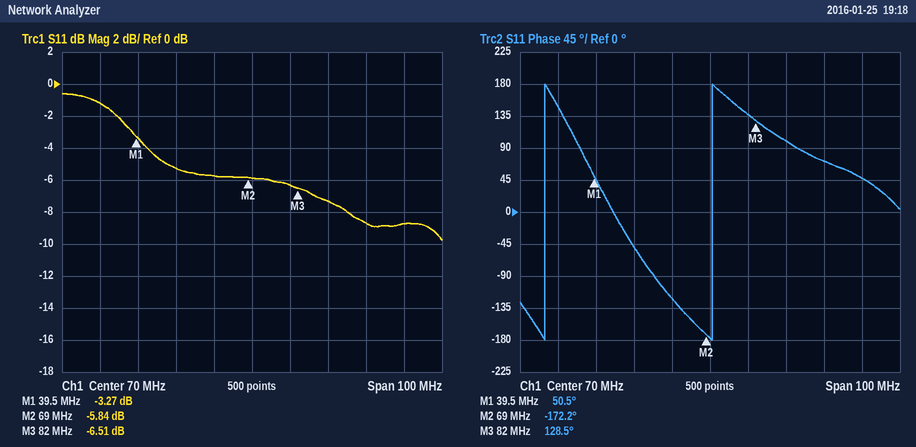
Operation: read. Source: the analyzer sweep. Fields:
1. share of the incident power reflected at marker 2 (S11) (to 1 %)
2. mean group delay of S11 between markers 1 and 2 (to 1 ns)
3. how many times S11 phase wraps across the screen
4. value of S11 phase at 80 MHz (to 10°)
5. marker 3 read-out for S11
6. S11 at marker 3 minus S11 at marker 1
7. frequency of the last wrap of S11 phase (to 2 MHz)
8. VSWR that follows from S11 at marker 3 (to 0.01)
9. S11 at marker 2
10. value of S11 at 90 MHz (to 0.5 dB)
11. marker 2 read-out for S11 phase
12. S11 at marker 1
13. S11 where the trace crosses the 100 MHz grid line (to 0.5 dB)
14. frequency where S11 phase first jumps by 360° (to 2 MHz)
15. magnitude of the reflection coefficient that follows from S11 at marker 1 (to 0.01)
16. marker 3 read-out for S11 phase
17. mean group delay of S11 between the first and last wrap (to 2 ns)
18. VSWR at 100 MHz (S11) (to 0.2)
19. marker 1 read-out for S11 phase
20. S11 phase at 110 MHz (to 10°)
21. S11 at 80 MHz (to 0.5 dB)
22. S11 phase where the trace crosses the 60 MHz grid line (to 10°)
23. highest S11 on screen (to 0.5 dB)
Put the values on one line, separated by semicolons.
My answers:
26 %; 21 ns; 2; 140°; -6.51 dB; -3.24 dB; 70 MHz; 2.79; -5.84 dB; -7.5 dB; -172.2°; -3.27 dB; -8.5 dB; 26 MHz; 0.69; 128.5°; 22 ns; 2.2; 50.5°; 50°; -6.5 dB; -120°; -0.5 dB
